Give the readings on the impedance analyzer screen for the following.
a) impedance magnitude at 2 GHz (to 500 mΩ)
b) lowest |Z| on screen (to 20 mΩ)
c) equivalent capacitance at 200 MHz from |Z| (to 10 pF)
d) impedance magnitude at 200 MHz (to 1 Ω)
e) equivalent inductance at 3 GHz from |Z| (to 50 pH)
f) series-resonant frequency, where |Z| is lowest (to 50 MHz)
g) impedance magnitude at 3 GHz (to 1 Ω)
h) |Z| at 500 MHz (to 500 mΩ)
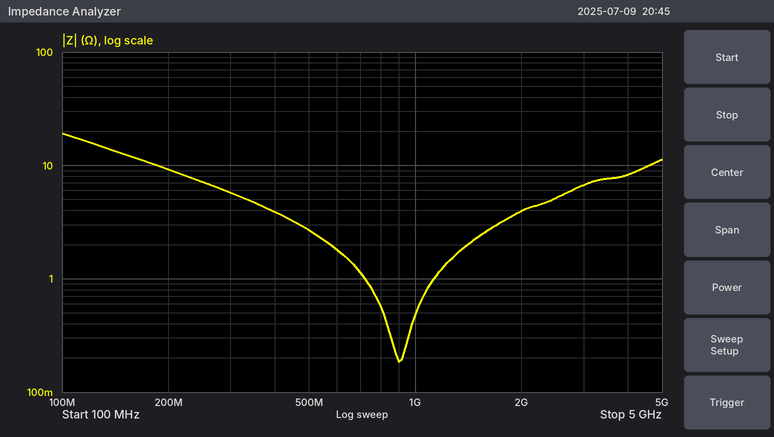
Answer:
4.0 Ω
180 mΩ
90 pF
9 Ω
350 pH
900 MHz
7 Ω
2.5 Ω
